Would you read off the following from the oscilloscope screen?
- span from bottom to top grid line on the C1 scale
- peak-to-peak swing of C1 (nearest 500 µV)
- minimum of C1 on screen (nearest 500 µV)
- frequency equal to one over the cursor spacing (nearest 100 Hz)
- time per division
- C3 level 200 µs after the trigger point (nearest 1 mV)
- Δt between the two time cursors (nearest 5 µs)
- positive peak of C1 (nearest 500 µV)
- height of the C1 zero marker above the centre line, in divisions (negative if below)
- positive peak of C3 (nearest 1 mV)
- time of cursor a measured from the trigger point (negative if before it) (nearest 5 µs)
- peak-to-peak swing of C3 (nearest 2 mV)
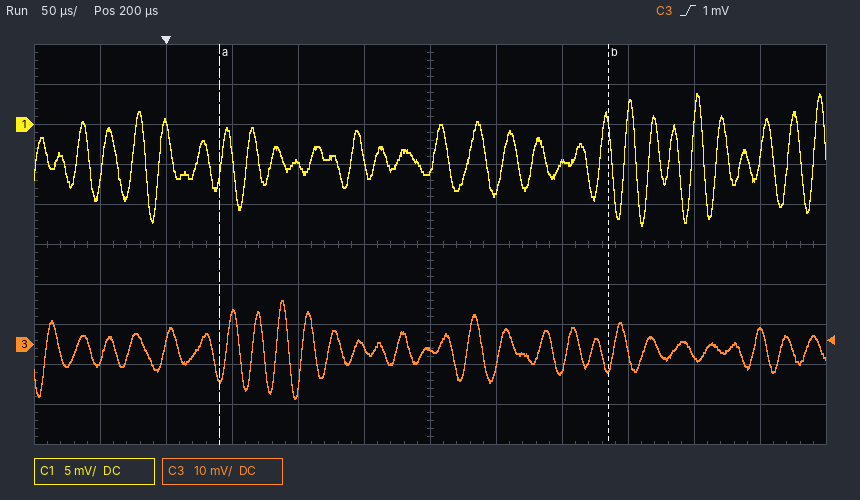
50 mV
16.5 mV
-12.5 mV
3.4 kHz
50 µs
-1 mV
295 µs
4.0 mV
+3.0 div
11 mV
+40 µs
24 mV
